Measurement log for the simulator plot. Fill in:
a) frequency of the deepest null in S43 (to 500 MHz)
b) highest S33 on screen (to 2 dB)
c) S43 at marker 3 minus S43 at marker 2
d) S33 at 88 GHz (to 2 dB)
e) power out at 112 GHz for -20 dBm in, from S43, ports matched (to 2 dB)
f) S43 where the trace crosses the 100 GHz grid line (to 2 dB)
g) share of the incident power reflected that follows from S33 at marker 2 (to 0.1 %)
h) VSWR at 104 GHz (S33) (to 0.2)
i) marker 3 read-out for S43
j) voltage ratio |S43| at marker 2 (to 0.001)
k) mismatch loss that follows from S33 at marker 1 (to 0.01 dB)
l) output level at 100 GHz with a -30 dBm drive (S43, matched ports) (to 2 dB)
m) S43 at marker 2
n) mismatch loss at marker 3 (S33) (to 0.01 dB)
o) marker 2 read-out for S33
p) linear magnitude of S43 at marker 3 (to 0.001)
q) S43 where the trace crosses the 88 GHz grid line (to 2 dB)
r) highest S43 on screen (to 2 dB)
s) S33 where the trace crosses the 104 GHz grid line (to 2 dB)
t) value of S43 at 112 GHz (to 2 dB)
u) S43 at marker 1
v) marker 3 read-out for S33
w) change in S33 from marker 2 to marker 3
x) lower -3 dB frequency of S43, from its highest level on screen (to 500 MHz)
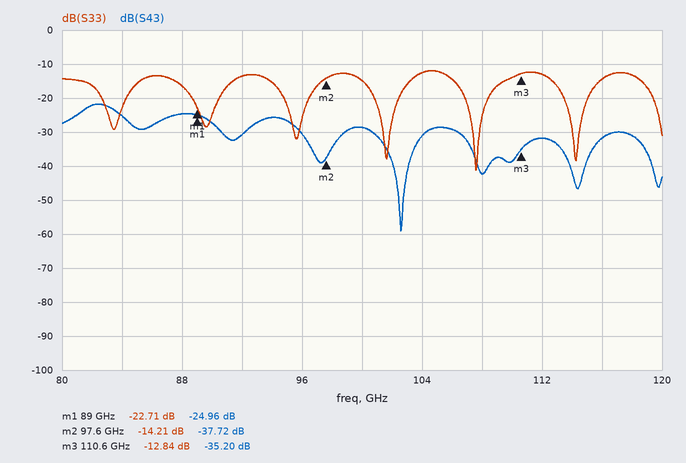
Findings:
102.5 GHz
-12 dB
2.52 dB
-16 dB
-52 dBm
-28 dB
3.8 %
1.6
-35.20 dB
0.013
0.02 dB
-58 dBm
-37.72 dB
0.23 dB
-14.21 dB
0.017
-24 dB
-22 dB
-12 dB
-32 dB
-24.96 dB
-12.84 dB
1.37 dB
81.0 GHz
